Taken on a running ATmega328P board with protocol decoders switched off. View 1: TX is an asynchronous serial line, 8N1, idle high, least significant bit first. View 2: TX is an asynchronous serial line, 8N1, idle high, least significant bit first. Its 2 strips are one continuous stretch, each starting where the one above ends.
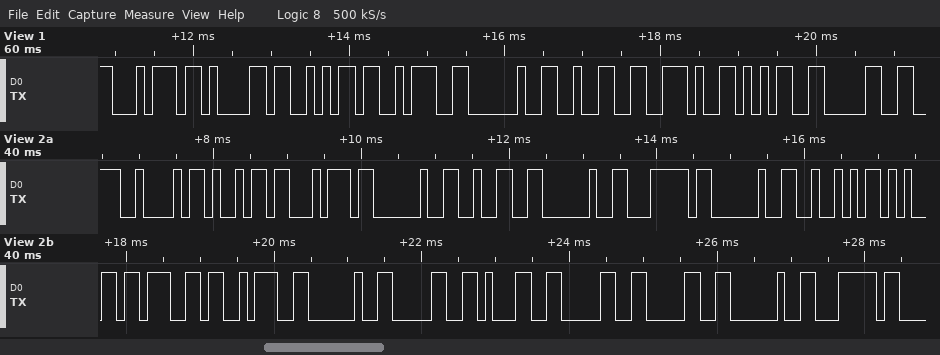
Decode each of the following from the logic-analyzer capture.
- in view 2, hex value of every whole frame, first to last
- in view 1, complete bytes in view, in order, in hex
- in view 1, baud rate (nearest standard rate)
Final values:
0x42 0x69 0x74 0x20 0x32 0x20 0x7C 0x20 0x52 0x65 0x67 0x3A 0x20 0x30 0x31 0x30 0x30 0x20 0x7C
74 61 6A 3A 20 32 2E 35 30
9600 baud
